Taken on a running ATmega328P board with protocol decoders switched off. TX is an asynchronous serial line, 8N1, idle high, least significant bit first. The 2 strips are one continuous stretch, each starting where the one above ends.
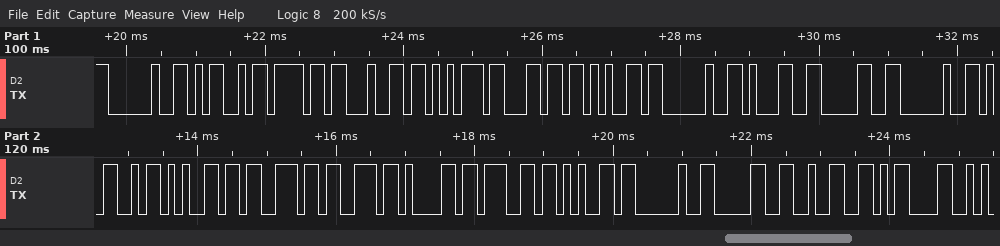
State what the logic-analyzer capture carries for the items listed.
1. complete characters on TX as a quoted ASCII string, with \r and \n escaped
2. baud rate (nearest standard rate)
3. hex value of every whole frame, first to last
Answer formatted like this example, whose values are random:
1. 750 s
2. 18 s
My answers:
1. " Module 10 Message 02\r"
2. 9600 baud
3. 20 4D 6F 64 75 6C 65 20 31 30 20 4D 65 73 73 61 67 65 20 30 32 0D
